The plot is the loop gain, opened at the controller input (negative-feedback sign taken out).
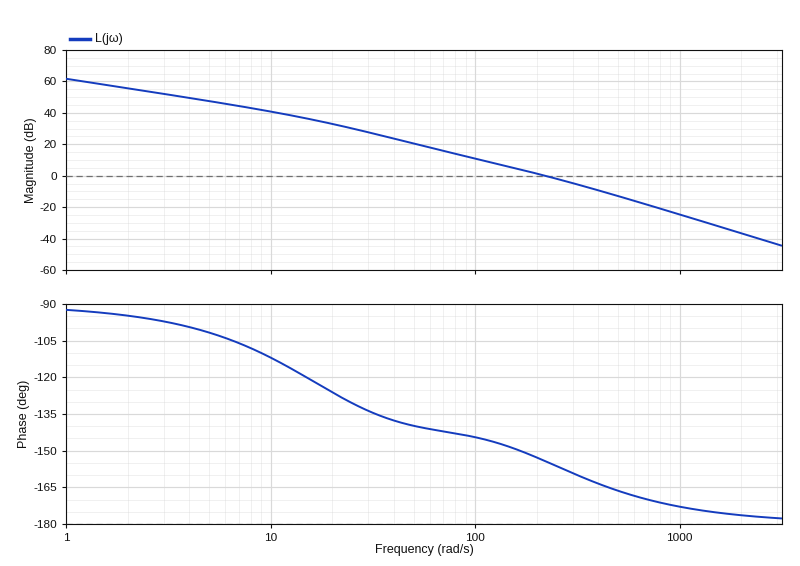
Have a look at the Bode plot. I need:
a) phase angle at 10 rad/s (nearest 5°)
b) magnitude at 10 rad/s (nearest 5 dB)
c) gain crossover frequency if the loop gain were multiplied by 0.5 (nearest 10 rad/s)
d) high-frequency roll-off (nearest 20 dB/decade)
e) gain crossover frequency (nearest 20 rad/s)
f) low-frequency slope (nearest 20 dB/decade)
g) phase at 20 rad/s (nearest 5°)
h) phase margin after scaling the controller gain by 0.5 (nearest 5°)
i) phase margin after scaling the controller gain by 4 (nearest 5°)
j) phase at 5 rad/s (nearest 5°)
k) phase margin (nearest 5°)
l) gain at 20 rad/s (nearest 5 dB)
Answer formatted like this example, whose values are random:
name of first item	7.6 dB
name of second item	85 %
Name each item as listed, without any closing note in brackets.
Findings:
phase angle at 10 rad/s	-110°
magnitude at 10 rad/s	40 dB
gain crossover frequency if the loop gain were multiplied by 0.5	140 rad/s
high-frequency roll-off	-40 dB/decade
gain crossover frequency	220 rad/s
low-frequency slope	-20 dB/decade
phase at 20 rad/s	-125°
phase margin after scaling the controller gain by 0.5	30°
phase margin after scaling the controller gain by 4	15°
phase at 5 rad/s	-100°
phase margin	25°
gain at 20 rad/s	35 dB
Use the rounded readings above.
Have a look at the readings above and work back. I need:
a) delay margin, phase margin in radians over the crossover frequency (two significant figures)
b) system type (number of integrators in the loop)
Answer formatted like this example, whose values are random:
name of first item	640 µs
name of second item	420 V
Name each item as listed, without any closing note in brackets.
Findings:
delay margin, phase margin in radians over the crossover frequency	0.0020 s
system type	1
